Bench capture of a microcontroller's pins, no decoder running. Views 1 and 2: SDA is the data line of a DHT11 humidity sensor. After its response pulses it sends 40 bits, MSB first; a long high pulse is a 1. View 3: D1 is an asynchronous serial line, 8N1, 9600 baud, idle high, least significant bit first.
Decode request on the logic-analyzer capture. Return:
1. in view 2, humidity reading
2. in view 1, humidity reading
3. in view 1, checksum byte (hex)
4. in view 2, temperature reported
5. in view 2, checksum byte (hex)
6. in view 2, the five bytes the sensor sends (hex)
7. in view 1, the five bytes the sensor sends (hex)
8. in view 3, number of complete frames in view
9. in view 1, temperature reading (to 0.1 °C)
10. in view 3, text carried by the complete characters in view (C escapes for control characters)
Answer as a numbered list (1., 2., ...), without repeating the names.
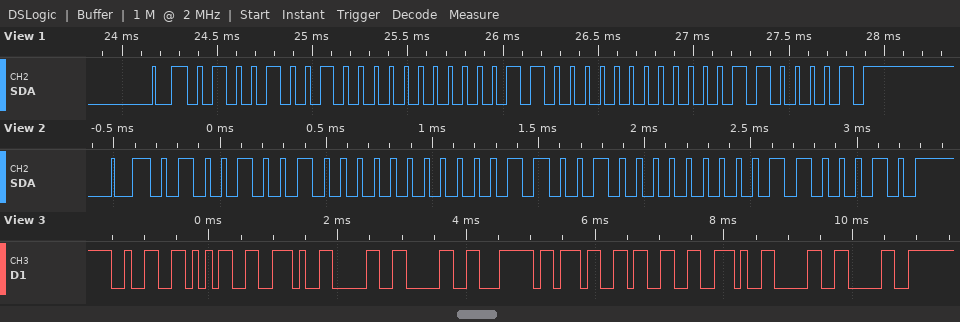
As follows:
1. 73 %
2. 73 %
3. 0x61
4. 25.0 °C
5. 0x62
6. 49 00 19 00 62
7. 49 00 18 00 61
8. 11
9. 24.0 °C
10. "25.00|73.00"
